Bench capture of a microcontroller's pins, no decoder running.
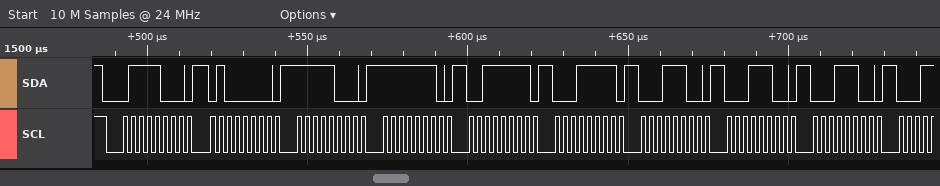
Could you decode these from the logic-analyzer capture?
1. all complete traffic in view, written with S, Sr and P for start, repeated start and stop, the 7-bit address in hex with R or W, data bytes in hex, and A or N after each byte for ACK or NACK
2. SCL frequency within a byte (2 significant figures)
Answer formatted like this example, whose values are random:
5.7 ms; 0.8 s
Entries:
S 3CW A 40 A F8 A FE A 3F A 1F A 1C A 1C A 1C A; 400 kHz
